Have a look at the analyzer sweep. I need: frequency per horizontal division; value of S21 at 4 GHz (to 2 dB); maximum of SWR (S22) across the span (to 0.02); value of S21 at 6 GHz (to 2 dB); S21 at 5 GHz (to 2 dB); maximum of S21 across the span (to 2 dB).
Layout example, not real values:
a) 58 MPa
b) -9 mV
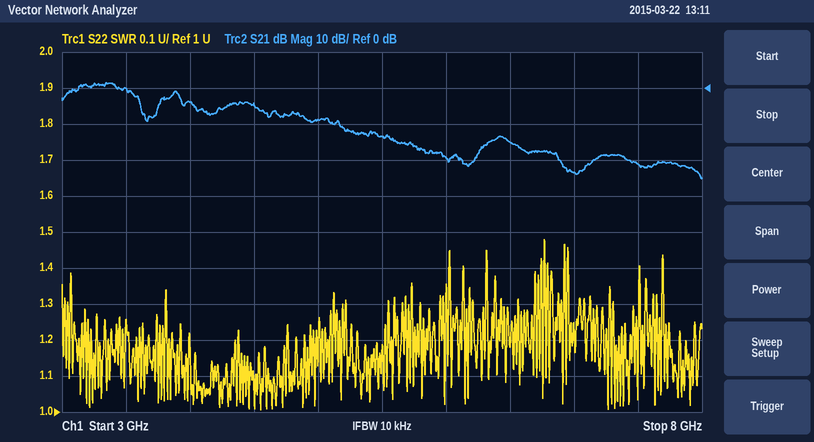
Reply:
a) 500 MHz
b) -4 dB
c) 1.48
d) -20 dB
e) -8 dB
f) 2 dB
